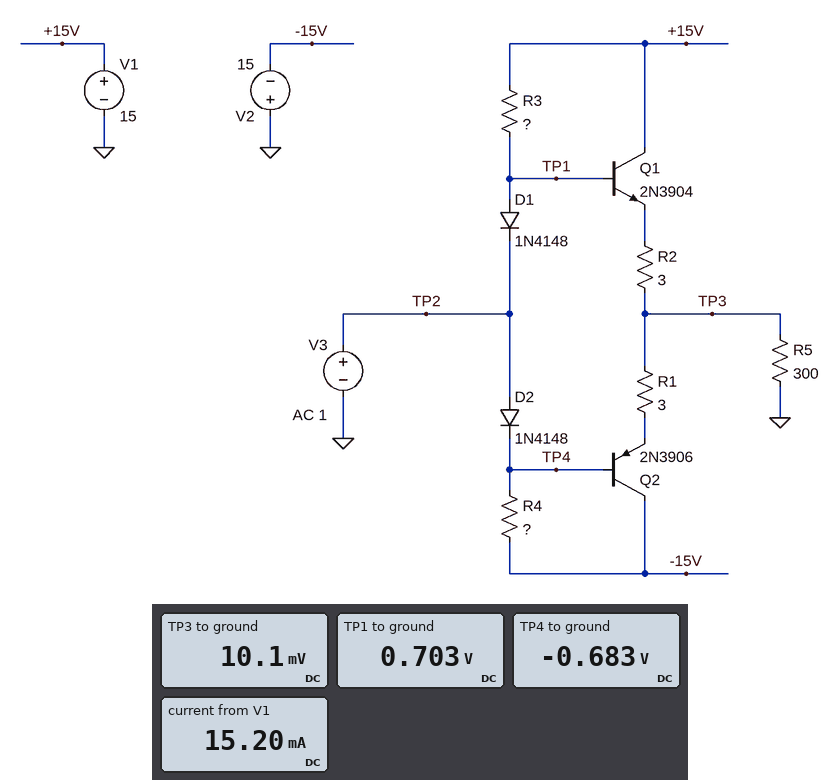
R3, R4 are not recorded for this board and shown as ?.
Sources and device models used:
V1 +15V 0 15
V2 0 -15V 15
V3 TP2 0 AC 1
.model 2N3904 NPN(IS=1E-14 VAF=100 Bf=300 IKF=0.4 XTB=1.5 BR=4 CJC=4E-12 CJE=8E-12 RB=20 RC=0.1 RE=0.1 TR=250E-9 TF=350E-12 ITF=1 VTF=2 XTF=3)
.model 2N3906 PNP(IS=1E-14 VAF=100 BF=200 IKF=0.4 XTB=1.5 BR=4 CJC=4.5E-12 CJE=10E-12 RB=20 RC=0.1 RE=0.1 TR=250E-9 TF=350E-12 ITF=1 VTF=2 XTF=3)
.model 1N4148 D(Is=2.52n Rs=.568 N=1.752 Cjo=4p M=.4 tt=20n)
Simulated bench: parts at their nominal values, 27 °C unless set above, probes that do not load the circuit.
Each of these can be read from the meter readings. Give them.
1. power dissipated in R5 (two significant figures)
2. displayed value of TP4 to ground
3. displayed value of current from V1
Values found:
340 nW
-0.683 V
15.20 mA
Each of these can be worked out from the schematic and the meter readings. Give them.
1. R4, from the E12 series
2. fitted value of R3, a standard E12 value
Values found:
1.8 kΩ
1.2 kΩ
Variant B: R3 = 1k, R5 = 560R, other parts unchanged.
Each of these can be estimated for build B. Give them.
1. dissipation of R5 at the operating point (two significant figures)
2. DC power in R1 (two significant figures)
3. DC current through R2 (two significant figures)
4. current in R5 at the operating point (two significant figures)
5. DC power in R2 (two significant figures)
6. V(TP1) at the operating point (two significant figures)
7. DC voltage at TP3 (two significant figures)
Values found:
400 nW
41 µW
3.7 mA
27 µA
42 µW
710 mV
15 mV
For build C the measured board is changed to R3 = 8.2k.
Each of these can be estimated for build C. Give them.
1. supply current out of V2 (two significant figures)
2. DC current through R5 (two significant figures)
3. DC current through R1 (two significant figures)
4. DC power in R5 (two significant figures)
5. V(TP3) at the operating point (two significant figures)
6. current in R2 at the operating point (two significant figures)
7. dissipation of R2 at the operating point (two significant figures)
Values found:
8.8 mA
110 µA
810 µA
3.8 µW
-34 mV
700 µA
1.5 µW
